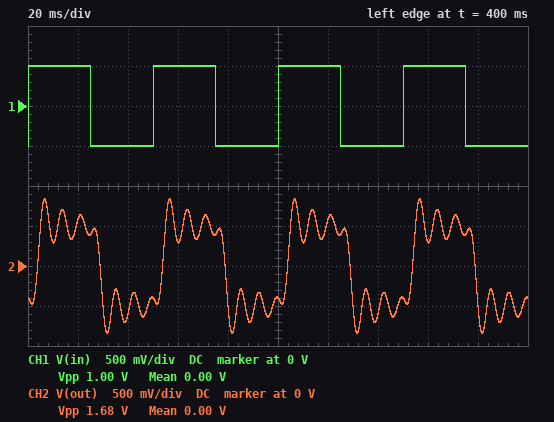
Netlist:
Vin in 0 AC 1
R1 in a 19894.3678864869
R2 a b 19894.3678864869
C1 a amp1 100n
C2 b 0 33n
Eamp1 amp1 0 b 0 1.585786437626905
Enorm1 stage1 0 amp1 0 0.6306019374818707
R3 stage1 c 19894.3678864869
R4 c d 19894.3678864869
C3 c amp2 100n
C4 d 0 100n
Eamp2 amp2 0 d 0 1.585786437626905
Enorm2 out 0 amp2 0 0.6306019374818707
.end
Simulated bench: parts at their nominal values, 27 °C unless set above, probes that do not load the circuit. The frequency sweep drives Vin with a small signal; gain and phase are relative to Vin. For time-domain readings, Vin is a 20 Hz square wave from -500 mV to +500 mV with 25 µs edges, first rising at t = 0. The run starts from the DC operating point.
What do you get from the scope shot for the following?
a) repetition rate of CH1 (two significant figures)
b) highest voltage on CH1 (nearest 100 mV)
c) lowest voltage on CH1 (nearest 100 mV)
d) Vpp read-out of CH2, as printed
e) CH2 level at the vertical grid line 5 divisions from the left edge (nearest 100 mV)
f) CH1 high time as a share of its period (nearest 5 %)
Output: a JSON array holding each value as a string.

["20 Hz", "500 mV", "-500 mV", "1.68 V", "-400 mV", "50 %"]
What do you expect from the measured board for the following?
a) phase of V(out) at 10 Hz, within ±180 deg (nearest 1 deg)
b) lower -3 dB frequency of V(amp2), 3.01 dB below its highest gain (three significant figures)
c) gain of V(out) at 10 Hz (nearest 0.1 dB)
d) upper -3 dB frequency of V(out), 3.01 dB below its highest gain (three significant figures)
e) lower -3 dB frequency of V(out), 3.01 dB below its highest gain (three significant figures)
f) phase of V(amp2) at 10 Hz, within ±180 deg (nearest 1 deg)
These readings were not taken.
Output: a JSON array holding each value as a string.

["-11 deg", "126 Hz", "0 dB", "146 Hz", "126 Hz", "-11 deg"]
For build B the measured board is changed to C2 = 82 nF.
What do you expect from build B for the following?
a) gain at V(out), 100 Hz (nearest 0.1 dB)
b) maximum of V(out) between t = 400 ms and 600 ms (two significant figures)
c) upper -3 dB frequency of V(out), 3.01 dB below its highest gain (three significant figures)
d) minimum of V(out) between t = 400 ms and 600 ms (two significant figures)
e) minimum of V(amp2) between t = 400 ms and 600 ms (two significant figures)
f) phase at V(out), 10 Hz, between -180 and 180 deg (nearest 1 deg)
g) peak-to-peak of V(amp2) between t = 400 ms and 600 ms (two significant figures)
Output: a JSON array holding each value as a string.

["-8.0 dB", "600 mV", "75.6 Hz", "-600 mV", "-960 mV", "-18 deg", "1.9 V"]
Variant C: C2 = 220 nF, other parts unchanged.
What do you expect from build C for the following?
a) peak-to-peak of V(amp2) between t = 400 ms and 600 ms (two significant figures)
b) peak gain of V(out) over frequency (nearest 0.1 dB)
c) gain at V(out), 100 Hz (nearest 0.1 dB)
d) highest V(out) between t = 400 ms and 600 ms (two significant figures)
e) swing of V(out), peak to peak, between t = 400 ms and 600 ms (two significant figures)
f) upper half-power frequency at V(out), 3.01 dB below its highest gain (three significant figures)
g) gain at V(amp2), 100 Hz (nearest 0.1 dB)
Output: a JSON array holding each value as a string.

["1.5 V", "0 dB", "-19.9 dB", "470 mV", "940 mV", "24.4 Hz", "-15.9 dB"]
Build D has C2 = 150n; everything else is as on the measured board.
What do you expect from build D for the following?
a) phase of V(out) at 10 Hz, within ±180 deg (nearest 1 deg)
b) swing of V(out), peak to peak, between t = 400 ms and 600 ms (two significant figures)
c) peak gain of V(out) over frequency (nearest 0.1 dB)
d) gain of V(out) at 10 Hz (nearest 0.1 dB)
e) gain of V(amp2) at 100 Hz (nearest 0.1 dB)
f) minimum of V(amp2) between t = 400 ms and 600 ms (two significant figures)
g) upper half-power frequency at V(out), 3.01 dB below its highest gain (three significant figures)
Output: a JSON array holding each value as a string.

["-27 deg", "1.0 V", "0 dB", "-0.2 dB", "-11.7 dB", "-790 mV", "40.6 Hz"]
